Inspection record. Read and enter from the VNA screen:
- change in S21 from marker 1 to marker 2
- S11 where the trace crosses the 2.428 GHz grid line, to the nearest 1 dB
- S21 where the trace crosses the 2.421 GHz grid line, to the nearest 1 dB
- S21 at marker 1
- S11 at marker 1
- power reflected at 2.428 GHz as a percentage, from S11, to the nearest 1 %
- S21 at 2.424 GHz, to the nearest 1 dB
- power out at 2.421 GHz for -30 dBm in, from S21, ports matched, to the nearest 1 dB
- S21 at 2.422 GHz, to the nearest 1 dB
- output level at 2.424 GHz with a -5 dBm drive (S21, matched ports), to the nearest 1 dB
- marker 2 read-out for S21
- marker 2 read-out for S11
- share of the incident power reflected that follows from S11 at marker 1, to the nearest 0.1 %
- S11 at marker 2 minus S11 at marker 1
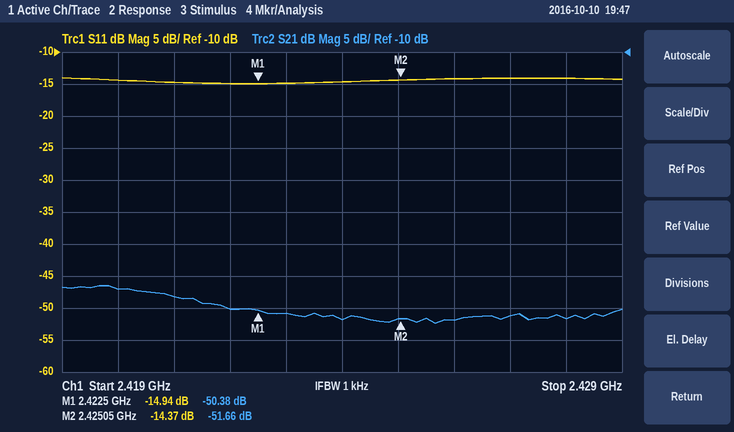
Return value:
-1.28 dB
-14 dB
-48 dB
-50.38 dB
-14.94 dB
4 %
-52 dB
-78 dBm
-50 dB
-57 dBm
-51.66 dB
-14.37 dB
3.2 %
0.57 dB
